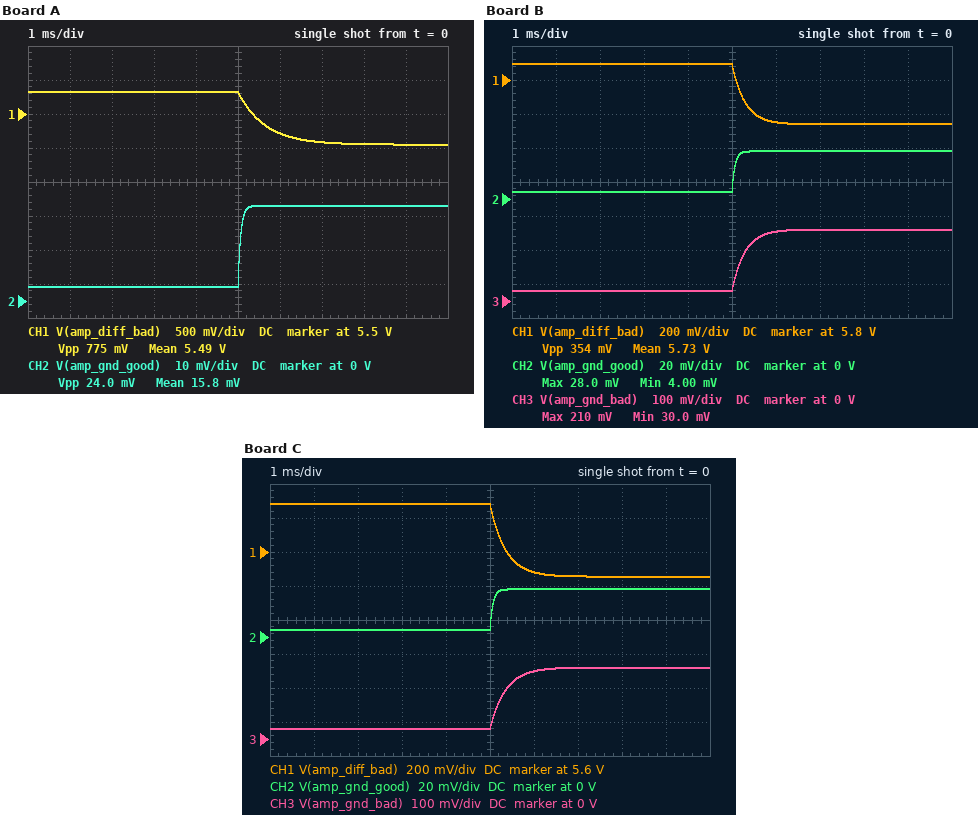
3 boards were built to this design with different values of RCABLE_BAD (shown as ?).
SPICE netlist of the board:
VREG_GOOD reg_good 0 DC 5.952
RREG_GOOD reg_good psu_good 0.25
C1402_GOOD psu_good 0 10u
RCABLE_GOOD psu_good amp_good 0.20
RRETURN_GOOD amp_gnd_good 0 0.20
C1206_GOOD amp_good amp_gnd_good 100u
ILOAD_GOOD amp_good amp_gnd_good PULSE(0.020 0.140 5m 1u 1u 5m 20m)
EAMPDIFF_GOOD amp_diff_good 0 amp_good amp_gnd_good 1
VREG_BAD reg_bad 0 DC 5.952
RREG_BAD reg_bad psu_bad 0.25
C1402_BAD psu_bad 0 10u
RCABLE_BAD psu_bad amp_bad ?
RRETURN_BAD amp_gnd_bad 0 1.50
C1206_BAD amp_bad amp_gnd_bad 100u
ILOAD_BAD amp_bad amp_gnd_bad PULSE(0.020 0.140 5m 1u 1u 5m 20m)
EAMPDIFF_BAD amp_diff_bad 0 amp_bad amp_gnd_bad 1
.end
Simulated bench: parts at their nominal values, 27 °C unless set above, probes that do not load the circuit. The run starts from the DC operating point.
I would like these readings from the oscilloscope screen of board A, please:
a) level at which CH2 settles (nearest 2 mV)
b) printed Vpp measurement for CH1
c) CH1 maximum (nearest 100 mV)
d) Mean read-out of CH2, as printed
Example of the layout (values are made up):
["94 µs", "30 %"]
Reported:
["28 mV", "775 mV", "5.8 V", "15.8 mV"]
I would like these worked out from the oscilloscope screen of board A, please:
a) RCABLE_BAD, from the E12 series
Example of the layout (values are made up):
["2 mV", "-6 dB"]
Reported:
["4.7 Ω"]
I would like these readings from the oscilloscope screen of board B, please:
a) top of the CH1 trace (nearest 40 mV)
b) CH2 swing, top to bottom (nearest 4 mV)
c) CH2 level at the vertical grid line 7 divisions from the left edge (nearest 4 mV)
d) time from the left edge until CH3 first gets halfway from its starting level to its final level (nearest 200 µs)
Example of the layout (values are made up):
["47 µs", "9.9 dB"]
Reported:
["5.88 V", "24 mV", "28 mV", "5.2 ms"]
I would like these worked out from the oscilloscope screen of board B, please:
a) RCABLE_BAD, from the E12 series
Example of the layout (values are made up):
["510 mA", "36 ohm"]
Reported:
["1.2 Ω"]
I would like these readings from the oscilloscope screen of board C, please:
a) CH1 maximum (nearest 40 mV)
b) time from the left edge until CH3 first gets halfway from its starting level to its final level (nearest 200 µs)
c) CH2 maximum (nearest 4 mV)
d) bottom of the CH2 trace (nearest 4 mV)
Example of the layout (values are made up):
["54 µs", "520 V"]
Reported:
["5.88 V", "5.2 ms", "28 mV", "4 mV"]
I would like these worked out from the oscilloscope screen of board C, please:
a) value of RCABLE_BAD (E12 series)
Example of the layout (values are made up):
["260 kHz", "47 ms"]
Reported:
["1.8 Ω"]
